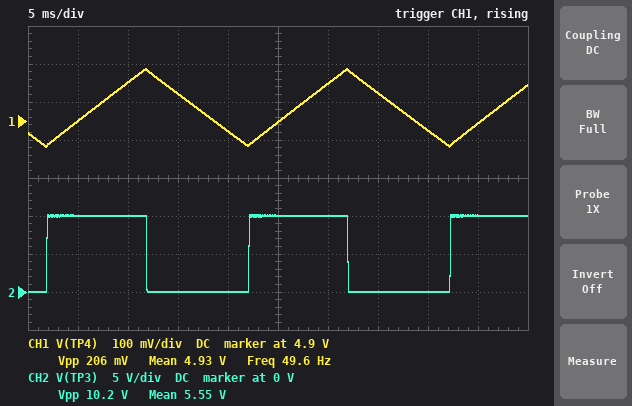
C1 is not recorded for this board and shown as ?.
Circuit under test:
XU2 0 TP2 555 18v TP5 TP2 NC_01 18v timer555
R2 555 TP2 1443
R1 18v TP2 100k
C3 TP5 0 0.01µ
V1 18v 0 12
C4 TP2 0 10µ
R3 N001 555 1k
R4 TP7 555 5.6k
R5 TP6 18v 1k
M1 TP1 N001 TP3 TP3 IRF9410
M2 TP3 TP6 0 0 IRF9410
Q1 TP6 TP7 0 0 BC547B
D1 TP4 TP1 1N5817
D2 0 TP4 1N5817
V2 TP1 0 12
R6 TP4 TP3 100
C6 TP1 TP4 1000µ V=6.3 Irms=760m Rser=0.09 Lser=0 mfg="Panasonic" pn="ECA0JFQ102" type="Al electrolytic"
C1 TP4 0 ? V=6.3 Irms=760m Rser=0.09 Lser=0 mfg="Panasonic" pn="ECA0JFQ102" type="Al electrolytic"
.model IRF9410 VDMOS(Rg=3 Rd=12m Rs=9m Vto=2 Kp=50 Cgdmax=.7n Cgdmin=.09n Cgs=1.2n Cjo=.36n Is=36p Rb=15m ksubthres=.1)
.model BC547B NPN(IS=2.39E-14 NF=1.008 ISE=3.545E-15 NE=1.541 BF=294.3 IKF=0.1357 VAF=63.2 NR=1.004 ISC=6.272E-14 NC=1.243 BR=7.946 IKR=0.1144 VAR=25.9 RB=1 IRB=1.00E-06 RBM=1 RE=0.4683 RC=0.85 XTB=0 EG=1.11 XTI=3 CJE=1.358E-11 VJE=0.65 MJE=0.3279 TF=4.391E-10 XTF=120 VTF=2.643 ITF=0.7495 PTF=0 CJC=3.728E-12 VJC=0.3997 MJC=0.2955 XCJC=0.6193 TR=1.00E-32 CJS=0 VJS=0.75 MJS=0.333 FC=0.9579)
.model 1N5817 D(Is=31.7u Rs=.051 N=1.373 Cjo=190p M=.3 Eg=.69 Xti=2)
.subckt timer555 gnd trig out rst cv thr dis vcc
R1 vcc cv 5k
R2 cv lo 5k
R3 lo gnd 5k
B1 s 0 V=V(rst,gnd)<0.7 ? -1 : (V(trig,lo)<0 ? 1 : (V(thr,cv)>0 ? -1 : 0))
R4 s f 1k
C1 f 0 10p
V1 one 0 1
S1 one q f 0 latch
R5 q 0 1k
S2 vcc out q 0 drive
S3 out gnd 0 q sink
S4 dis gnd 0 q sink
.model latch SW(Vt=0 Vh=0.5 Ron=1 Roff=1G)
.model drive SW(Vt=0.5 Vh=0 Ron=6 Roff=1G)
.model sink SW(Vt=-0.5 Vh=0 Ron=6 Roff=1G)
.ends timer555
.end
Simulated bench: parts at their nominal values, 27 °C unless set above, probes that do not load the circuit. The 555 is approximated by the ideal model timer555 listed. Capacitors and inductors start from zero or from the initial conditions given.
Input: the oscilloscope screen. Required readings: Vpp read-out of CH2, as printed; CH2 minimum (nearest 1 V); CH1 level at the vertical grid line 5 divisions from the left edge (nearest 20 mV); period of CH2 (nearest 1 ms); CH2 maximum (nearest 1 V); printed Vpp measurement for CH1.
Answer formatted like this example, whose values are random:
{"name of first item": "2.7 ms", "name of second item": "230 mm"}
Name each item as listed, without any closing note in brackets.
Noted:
{"Vpp read-out of CH2, as printed": "10.2 V", "CH2 minimum": "0 V", "CH1 level at the vertical grid line 5 divisions from the left edge": "4.90 V", "period of CH2": "20 ms", "CH2 maximum": "10 V", "printed Vpp measurement for CH1": "206 mV"}
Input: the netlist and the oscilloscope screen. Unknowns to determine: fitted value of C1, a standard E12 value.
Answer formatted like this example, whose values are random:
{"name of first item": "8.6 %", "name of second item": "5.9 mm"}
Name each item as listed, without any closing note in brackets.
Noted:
{"fitted value of C1, a standard E12 value": "1.5 mF"}
